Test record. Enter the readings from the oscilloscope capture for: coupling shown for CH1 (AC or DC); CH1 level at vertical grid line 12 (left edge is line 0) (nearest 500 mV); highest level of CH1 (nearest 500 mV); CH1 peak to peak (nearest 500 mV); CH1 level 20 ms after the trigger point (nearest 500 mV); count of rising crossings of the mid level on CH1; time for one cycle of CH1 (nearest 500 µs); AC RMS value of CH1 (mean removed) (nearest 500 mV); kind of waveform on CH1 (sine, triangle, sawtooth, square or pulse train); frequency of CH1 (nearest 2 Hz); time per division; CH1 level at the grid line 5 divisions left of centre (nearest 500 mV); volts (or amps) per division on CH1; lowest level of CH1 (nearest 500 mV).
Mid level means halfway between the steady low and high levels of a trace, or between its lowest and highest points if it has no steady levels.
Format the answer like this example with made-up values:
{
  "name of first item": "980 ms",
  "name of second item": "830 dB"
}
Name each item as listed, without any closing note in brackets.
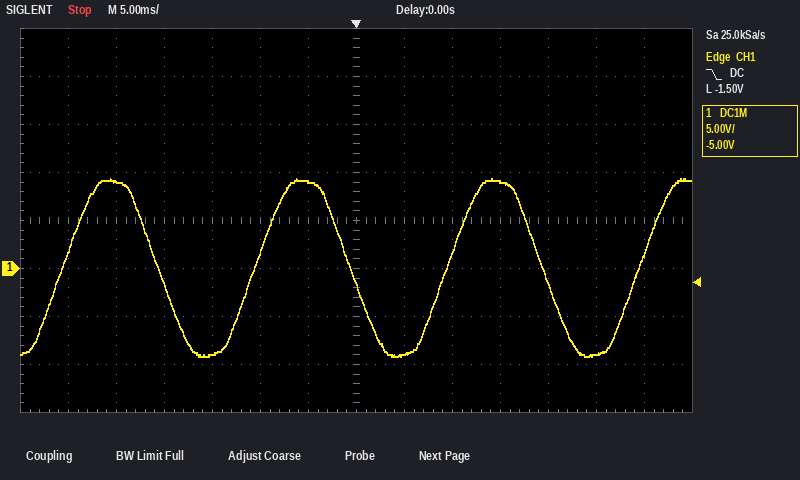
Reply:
{
  "coupling shown for CH1": "DC",
  "CH1 level at vertical grid line 12 (left edge is line 0)": "-9.0 V",
  "highest level of CH1": "9.5 V",
  "CH1 peak to peak": "18.5 V",
  "CH1 level 20 ms after the trigger point": "-1.5 V",
  "count of rising crossings of the mid level on CH1": "4",
  "time for one cycle of CH1": "20.0 ms",
  "AC RMS value of CH1 (mean removed)": "6.5 V",
  "kind of waveform on CH1": "sine",
  "frequency of CH1": "50 Hz",
  "time per division": "5 ms",
  "CH1 level at the grid line 5 divisions left of centre": "9.0 V",
  "volts (or amps) per division on CH1": "5 V",
  "lowest level of CH1": "-9.0 V"
}
